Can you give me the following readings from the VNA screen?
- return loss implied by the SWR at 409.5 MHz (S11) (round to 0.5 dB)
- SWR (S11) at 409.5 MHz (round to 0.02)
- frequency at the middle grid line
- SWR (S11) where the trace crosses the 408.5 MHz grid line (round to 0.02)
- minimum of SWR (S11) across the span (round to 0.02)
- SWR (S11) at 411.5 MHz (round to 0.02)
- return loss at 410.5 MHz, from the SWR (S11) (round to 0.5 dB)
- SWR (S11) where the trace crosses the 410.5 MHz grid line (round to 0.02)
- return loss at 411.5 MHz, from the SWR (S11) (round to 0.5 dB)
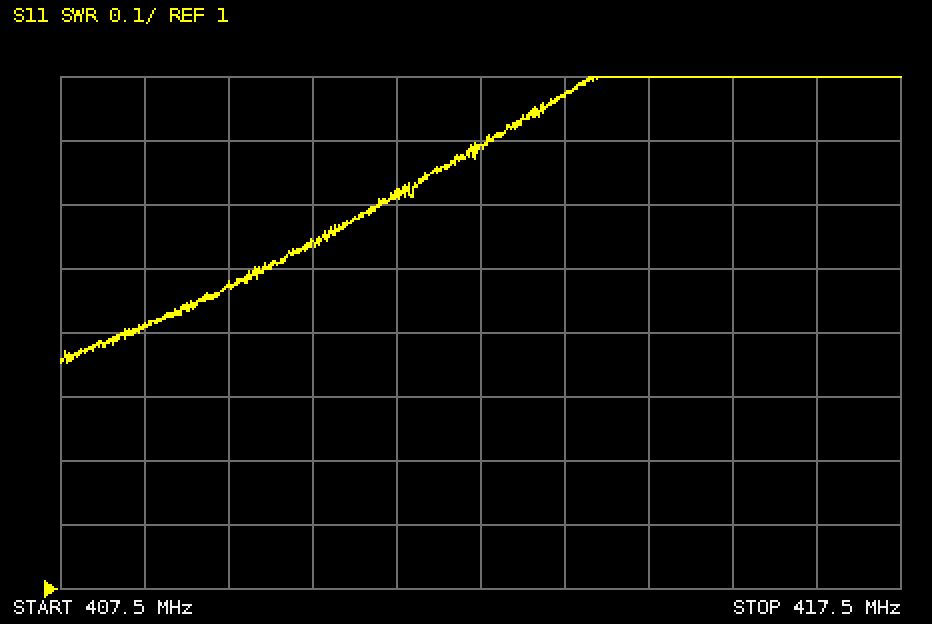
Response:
14.5 dB
1.48
412.5 MHz
1.42
1.36
1.62
13.5 dB
1.54
12.5 dB
